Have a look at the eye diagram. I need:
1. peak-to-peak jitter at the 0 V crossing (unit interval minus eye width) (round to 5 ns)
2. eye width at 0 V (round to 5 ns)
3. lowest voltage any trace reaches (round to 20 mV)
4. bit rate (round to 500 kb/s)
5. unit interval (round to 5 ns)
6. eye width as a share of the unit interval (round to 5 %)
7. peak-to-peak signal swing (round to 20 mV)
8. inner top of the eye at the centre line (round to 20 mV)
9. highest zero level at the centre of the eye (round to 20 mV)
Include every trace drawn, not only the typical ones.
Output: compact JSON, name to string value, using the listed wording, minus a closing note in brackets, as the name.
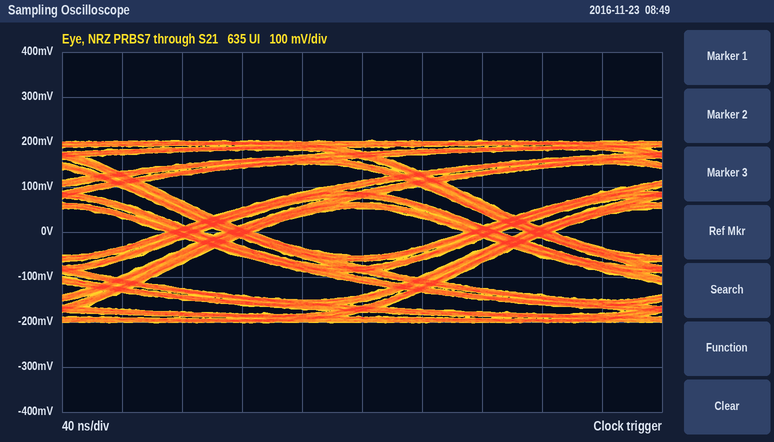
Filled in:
{"peak-to-peak jitter at the 0 V crossing (unit interval minus eye width)": "60 ns", "eye width at 0 V": "140 ns", "lowest voltage any trace reaches": "-200 mV", "bit rate": "5.0 Mb/s", "unit interval": "200 ns", "eye width as a share of the unit interval": "70 %", "peak-to-peak signal swing": "400 mV", "inner top of the eye at the centre line": "60 mV", "highest zero level at the centre of the eye": "-60 mV"}
